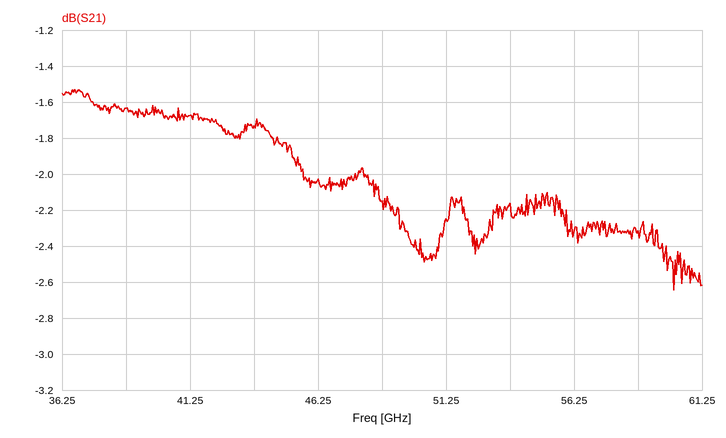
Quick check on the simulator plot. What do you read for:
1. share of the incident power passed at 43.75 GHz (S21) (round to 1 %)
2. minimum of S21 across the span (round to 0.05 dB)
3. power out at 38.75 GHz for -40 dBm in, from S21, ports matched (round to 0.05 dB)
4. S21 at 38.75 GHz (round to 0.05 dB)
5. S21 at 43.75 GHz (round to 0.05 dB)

67 %
-2.65 dB
-41.65 dBm
-1.65 dB
-1.75 dB
